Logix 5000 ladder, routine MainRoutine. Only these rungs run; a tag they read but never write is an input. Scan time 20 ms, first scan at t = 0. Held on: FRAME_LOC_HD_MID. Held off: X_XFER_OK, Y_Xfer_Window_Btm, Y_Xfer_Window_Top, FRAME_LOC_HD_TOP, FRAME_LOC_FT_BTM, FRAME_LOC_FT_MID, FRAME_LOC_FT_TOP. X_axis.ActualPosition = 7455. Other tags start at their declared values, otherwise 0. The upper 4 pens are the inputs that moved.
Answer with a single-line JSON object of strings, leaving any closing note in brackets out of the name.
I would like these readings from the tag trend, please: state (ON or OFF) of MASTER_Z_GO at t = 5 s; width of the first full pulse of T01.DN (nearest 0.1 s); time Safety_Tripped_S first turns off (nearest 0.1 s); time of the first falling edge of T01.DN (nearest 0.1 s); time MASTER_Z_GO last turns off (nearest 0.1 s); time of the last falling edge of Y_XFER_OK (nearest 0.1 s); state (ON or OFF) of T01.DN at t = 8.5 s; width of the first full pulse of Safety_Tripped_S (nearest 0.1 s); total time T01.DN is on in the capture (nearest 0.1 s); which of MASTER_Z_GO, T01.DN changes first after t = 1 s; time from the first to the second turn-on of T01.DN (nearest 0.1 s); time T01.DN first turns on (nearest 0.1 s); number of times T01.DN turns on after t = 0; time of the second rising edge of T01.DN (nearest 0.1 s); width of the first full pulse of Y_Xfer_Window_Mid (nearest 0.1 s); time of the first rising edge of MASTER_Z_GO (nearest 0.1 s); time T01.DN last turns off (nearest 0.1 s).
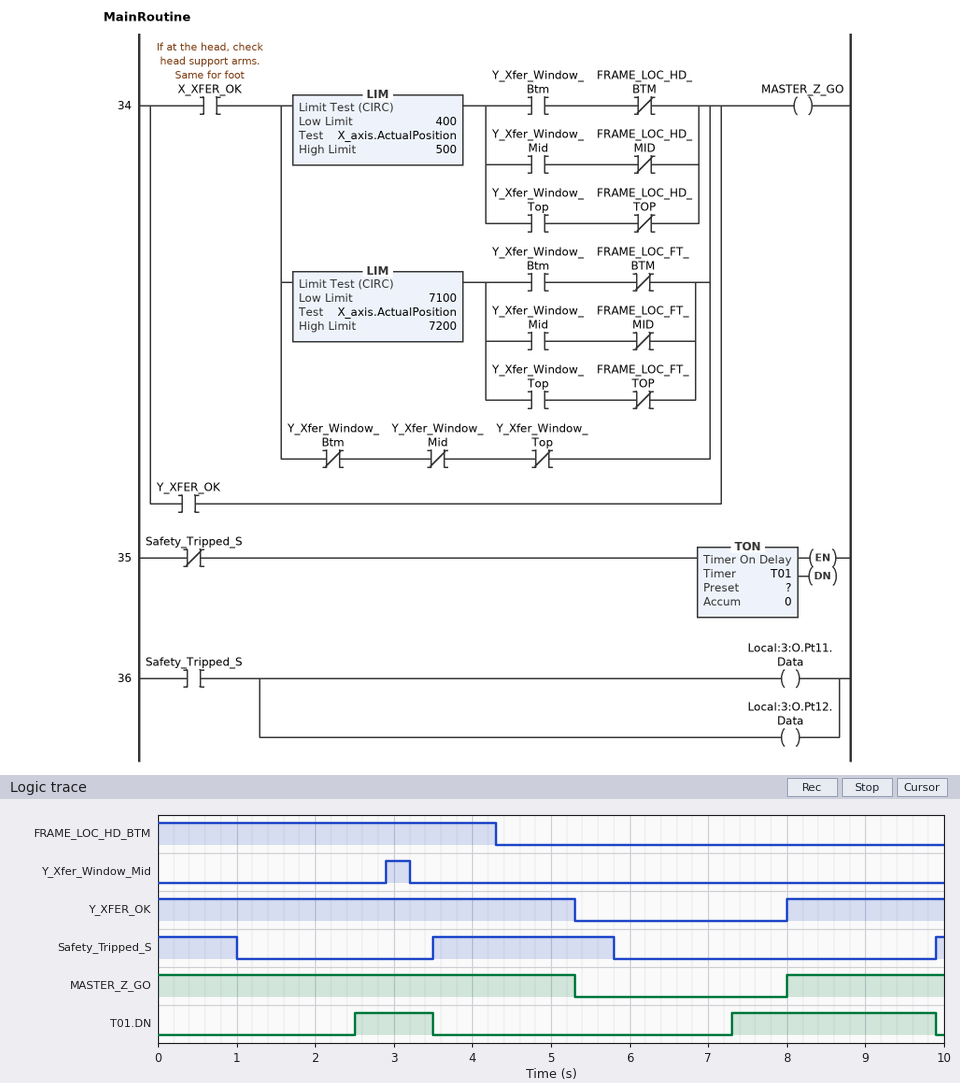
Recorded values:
{"state (ON or OFF) of MASTER_Z_GO at t = 5 s": "ON", "width of the first full pulse of T01.DN": "1.0 s", "time Safety_Tripped_S first turns off": "1.0 s", "time of the first falling edge of T01.DN": "3.5 s", "time MASTER_Z_GO last turns off": "5.3 s", "time of the last falling edge of Y_XFER_OK": "5.3 s", "state (ON or OFF) of T01.DN at t = 8.5 s": "ON", "width of the first full pulse of Safety_Tripped_S": "2.3 s", "total time T01.DN is on in the capture": "3.6 s", "which of MASTER_Z_GO, T01.DN changes first after t = 1 s": "T01.DN", "time from the first to the second turn-on of T01.DN": "4.8 s", "time T01.DN first turns on": "2.5 s", "number of times T01.DN turns on after t = 0": "2", "time of the second rising edge of T01.DN": "7.3 s", "width of the first full pulse of Y_Xfer_Window_Mid": "0.3 s", "time of the first rising edge of MASTER_Z_GO": "8.0 s", "time T01.DN last turns off": "9.9 s"}
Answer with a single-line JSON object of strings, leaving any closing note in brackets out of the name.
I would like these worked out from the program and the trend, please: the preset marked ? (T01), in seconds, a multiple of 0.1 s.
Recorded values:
{"the preset marked ? (T01), in seconds, a multiple of 0.1 s": "1.5 s"}
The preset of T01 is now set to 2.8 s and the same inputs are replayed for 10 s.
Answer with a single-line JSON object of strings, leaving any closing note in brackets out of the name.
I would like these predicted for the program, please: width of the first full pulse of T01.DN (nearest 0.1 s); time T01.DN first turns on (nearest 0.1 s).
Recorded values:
{"width of the first full pulse of T01.DN": "1.3 s", "time T01.DN first turns on": "8.6 s"}
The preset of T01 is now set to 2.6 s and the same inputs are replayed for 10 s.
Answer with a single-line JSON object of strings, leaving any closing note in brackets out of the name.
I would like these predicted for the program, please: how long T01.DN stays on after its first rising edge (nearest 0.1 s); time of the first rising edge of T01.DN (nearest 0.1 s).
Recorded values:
{"how long T01.DN stays on after its first rising edge": "1.5 s", "time of the first rising edge of T01.DN": "8.4 s"}
